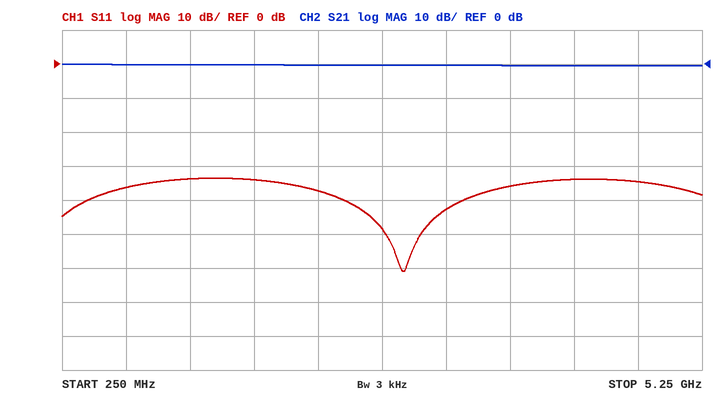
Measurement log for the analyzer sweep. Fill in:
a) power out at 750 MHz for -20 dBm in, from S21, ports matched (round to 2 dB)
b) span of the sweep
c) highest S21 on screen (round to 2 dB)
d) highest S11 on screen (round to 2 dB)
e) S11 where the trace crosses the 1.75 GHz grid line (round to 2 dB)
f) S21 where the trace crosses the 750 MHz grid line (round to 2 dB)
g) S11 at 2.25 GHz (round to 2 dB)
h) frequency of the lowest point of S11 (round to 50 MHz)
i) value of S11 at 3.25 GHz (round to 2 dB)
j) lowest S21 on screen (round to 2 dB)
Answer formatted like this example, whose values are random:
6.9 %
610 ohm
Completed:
-20 dBm
5 GHz
0 dB
-34 dB
-34 dB
0 dB
-38 dB
2.90 GHz
-42 dB
0 dB
